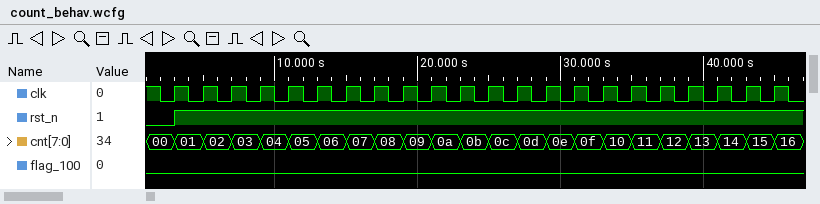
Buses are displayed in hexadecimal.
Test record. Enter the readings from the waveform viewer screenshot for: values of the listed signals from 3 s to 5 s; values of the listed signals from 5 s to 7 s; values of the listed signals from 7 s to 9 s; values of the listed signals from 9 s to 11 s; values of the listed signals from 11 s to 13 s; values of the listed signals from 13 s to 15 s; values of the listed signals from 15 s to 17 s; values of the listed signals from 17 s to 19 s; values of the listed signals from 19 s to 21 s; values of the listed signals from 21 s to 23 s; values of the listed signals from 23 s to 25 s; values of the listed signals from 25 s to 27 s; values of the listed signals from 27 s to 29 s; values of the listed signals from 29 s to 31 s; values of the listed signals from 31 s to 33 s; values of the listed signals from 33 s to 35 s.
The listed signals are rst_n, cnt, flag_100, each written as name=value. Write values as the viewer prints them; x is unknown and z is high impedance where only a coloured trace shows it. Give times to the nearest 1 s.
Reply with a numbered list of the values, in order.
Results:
1. rst_n=1, cnt=01, flag_100=0
2. rst_n=1, cnt=02, flag_100=0
3. rst_n=1, cnt=03, flag_100=0
4. rst_n=1, cnt=04, flag_100=0
5. rst_n=1, cnt=05, flag_100=0
6. rst_n=1, cnt=06, flag_100=0
7. rst_n=1, cnt=07, flag_100=0
8. rst_n=1, cnt=08, flag_100=0
9. rst_n=1, cnt=09, flag_100=0
10. rst_n=1, cnt=0a, flag_100=0
11. rst_n=1, cnt=0b, flag_100=0
12. rst_n=1, cnt=0c, flag_100=0
13. rst_n=1, cnt=0d, flag_100=0
14. rst_n=1, cnt=0e, flag_100=0
15. rst_n=1, cnt=0f, flag_100=0
16. rst_n=1, cnt=10, flag_100=0
